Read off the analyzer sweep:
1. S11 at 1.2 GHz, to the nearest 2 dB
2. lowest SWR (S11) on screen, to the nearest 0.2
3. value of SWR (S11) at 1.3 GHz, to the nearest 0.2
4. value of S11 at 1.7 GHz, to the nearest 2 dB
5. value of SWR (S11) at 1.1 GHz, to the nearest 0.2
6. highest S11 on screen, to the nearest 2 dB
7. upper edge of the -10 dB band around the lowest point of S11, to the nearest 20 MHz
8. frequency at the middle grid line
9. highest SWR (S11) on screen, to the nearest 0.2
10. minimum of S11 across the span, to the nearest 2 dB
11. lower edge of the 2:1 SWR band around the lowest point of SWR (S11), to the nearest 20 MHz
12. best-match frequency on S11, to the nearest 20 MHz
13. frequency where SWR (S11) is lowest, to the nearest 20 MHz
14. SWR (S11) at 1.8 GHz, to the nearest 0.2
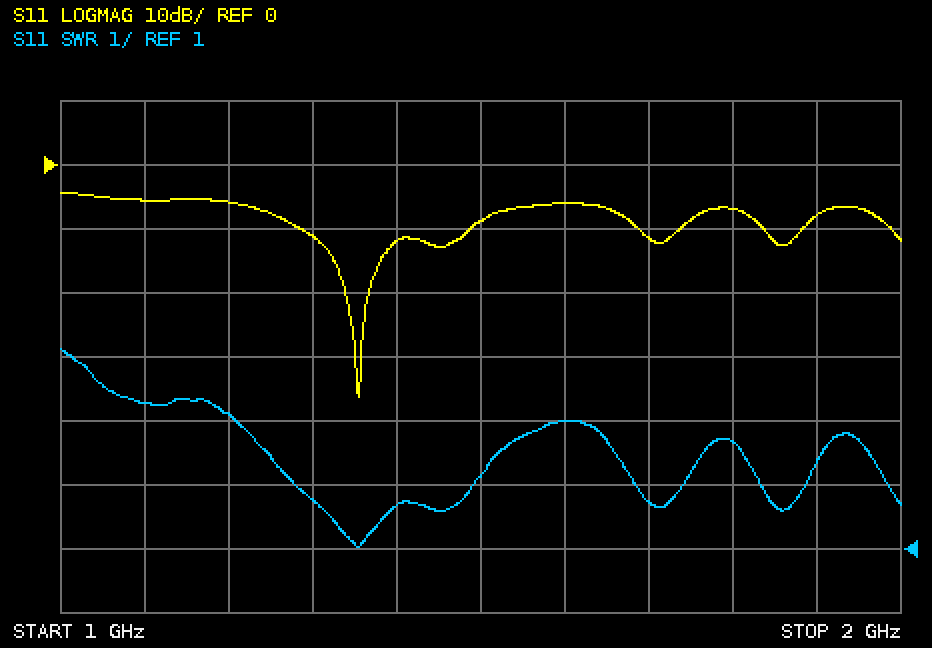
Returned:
-6 dB
1.0
1.8
-12 dB
3.2
-4 dB
1.48 GHz
1.5 GHz
4.2
-36 dB
1.28 GHz
1.36 GHz
1.36 GHz
2.6
